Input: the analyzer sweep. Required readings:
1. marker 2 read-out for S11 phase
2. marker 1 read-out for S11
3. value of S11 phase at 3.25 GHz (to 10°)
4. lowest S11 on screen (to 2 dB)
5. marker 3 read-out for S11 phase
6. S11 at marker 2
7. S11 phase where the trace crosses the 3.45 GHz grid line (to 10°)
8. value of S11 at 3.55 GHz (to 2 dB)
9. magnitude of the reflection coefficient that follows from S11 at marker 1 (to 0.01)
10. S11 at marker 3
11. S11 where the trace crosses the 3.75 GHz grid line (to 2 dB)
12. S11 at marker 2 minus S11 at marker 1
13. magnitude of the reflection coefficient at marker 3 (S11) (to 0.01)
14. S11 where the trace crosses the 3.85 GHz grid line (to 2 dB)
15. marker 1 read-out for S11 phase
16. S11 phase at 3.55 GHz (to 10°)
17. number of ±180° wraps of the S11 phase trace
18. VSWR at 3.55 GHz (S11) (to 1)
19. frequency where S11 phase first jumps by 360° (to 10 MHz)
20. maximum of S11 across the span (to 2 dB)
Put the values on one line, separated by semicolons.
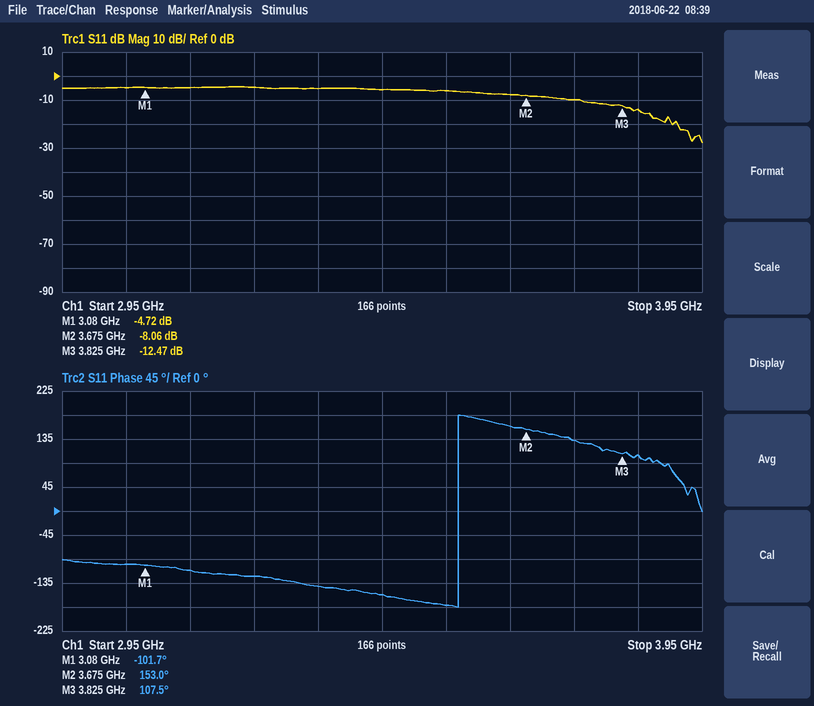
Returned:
153.0°; -4.72 dB; -120°; -28 dB; 107.5°; -8.06 dB; -160°; -6 dB; 0.58; -12.47 dB; -10 dB; -3.34 dB; 0.24; -14 dB; -101.7°; -180°; 1; 3; 3.57 GHz; -4 dB
